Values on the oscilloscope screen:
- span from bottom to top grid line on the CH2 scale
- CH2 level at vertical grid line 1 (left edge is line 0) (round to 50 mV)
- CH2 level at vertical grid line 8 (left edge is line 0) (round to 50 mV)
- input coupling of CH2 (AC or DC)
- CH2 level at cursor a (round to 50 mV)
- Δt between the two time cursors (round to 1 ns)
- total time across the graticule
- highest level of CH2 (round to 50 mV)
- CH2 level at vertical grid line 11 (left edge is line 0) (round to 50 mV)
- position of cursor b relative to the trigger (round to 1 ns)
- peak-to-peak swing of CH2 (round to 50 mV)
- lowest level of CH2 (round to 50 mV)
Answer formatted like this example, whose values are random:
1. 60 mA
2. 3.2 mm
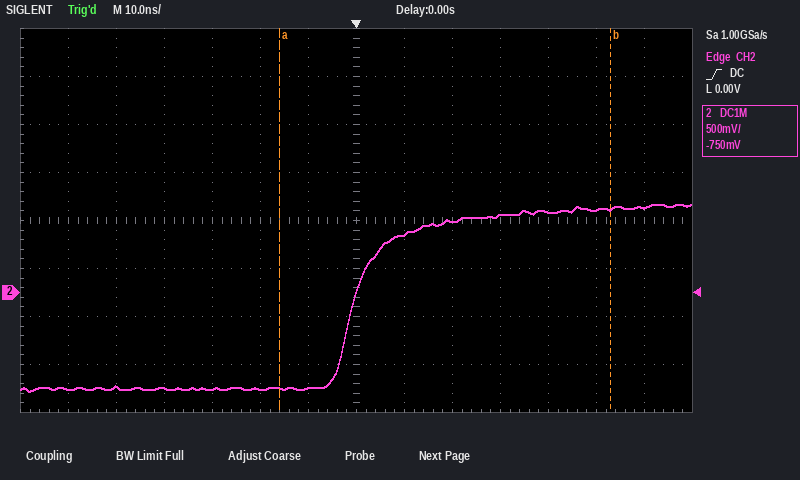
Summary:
1. 4 V
2. -1.00 V
3. 600 mV
4. DC
5. -1.00 V
6. 69 ns
7. 140 ns
8. 900 mV
9. 850 mV
10. +53 ns
11. 1.95 V
12. -1.05 V
